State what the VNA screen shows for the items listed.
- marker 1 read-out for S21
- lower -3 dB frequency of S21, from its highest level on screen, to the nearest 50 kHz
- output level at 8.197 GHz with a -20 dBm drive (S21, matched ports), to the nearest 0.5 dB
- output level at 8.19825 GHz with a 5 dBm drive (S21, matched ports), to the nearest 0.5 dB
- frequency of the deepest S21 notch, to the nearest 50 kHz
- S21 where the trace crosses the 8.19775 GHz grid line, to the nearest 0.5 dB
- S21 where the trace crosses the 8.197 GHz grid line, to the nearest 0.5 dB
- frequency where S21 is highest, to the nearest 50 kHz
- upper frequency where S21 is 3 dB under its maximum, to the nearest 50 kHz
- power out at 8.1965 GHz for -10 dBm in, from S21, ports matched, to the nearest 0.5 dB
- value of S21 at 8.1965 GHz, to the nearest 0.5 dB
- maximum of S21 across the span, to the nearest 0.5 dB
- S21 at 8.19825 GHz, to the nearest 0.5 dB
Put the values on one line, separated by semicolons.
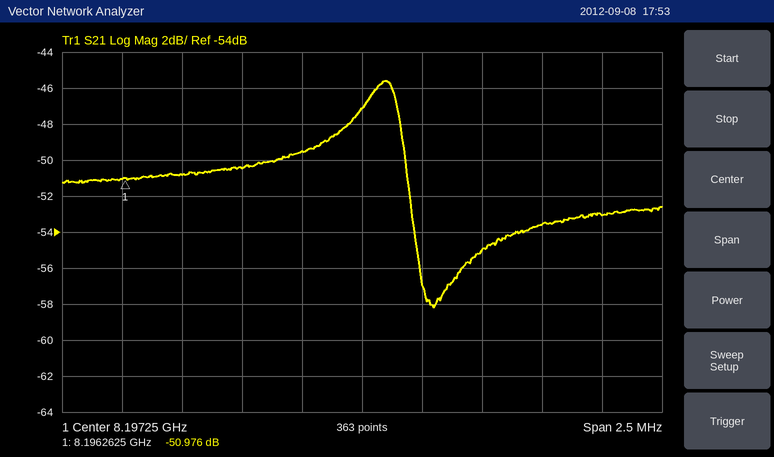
-50.976 dB; 8.19715 GHz; -69.5 dBm; -48.0 dBm; 8.19755 GHz; -55.0 dB; -49.5 dB; 8.19735 GHz; 8.19740 GHz; -61.0 dBm; -51.0 dB; -45.5 dB; -53.0 dB
